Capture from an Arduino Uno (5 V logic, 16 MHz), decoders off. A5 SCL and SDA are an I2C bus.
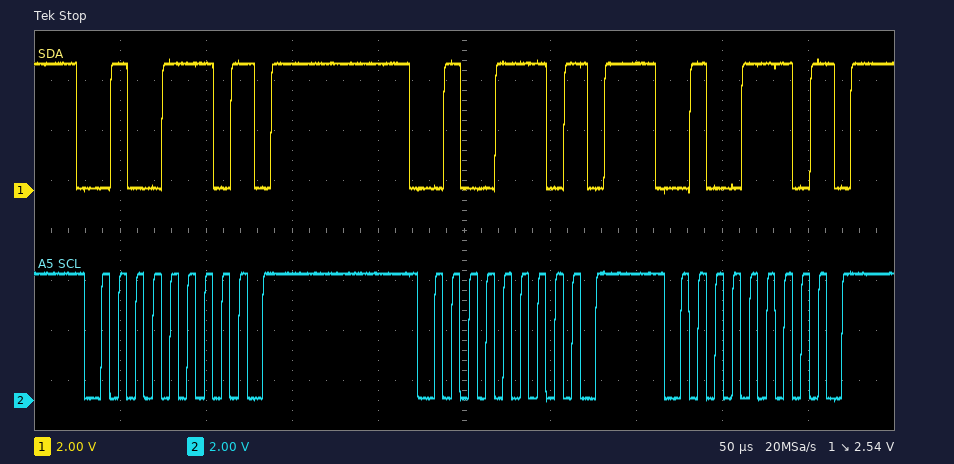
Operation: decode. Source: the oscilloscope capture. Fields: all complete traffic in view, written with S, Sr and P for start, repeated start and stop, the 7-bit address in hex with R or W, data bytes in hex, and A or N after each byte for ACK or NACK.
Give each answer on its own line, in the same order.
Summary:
S 27W N P S 27W N P S 27W N P
